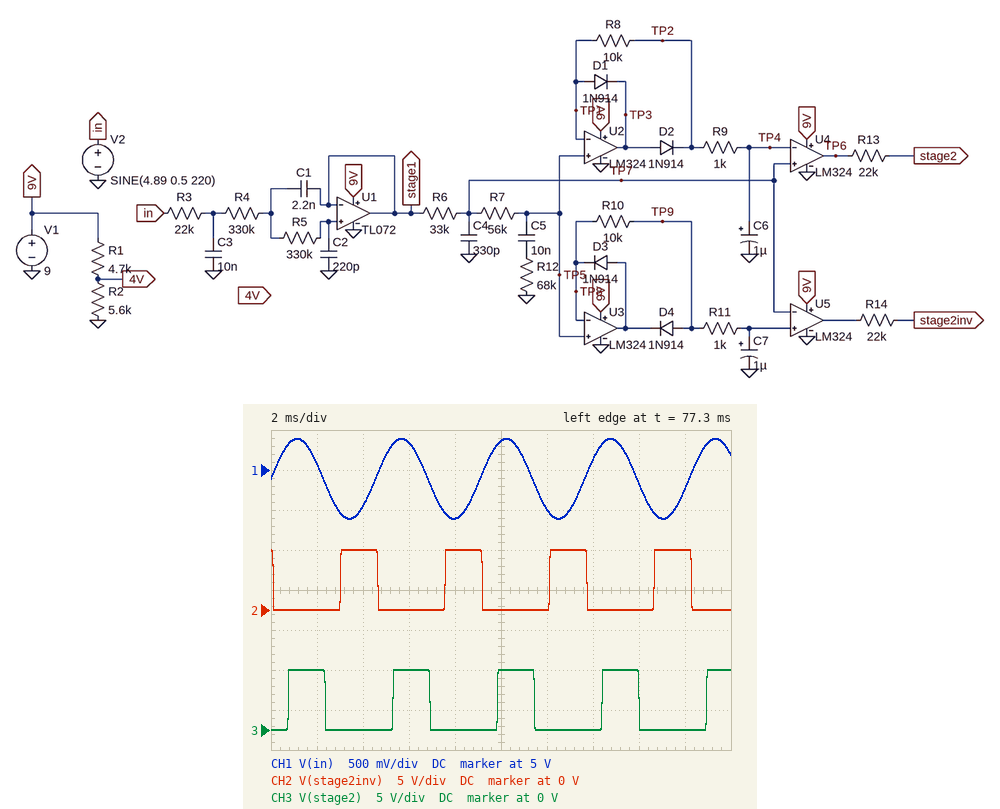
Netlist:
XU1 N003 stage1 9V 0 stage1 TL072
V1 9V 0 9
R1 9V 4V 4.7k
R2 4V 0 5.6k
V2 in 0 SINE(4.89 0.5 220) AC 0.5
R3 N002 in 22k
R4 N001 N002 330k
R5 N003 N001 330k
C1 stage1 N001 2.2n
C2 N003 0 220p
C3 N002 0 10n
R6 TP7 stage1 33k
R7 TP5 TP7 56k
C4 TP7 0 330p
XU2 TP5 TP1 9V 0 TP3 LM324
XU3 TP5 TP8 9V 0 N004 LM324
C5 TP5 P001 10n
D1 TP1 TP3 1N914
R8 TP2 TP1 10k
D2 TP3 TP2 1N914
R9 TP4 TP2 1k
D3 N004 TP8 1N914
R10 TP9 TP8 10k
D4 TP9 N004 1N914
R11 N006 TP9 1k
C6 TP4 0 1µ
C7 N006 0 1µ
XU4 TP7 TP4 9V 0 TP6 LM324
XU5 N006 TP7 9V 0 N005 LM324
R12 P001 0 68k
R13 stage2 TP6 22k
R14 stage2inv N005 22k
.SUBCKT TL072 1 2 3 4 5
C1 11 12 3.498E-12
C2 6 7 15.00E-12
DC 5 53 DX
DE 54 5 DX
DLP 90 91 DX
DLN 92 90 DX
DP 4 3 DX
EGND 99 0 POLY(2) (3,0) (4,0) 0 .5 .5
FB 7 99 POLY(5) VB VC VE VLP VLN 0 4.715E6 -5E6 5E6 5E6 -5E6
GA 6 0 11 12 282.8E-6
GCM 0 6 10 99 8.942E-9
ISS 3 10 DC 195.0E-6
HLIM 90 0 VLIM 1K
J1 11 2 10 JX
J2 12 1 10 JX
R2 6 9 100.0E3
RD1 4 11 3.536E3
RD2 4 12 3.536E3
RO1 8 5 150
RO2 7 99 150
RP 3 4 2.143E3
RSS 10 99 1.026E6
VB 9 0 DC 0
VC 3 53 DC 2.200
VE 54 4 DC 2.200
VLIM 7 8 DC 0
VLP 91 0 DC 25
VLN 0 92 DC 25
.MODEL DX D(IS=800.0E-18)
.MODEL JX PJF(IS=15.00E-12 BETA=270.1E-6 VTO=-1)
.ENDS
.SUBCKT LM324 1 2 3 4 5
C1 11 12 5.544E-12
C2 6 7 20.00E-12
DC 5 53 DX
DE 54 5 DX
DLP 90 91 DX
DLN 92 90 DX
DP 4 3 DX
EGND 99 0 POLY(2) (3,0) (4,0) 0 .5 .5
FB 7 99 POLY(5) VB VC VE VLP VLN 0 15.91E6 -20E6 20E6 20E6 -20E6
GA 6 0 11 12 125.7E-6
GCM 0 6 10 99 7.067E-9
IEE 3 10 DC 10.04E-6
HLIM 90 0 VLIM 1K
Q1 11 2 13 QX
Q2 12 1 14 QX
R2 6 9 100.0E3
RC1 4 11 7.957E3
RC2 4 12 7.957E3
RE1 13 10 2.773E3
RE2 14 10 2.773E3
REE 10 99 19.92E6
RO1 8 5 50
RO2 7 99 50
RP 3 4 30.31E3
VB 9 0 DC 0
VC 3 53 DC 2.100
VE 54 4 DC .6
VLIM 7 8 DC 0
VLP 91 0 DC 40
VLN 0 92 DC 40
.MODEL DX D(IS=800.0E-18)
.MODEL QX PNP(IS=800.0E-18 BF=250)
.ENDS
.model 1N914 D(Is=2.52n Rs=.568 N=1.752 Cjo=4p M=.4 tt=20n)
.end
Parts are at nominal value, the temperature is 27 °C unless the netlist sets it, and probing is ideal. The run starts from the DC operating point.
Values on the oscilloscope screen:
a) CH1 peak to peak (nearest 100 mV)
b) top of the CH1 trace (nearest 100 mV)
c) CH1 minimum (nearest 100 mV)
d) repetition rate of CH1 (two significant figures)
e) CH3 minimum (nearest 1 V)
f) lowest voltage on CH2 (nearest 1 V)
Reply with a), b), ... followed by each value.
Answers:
a) 1.0 V
b) 5.4 V
c) 4.4 V
d) 220 Hz
e) 0 V
f) 0 V
